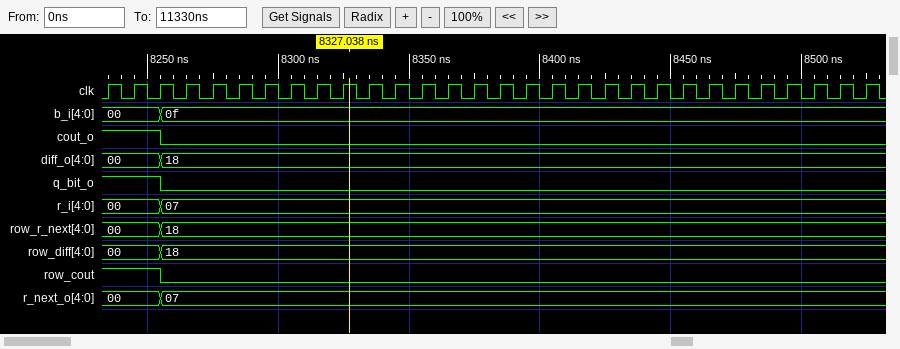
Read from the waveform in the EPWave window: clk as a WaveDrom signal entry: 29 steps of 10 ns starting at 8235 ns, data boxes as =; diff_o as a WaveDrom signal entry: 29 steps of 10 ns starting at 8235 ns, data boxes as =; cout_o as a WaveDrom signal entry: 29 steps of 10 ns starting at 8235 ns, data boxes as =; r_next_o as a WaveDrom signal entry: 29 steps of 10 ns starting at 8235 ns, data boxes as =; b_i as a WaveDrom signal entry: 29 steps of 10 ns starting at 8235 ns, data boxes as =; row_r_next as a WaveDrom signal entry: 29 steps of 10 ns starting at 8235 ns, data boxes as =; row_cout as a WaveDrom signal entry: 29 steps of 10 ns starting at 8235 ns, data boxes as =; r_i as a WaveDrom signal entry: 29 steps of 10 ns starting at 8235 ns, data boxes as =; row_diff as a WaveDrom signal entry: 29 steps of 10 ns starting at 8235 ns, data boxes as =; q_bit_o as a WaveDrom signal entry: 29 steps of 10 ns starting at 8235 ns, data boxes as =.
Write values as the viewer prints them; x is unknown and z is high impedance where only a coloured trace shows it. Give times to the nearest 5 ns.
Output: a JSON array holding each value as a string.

["{name: 'clk', wave: 'p............................'}", "{name: 'diff_o', wave: '=.=..........................', data: '00 18'}", "{name: 'cout_o', wave: '1.0..........................'}", "{name: 'r_next_o', wave: '=.=..........................', data: '00 07'}", "{name: 'b_i', wave: '=.=..........................', data: '00 0f'}", "{name: 'row_r_next', wave: '=.=..........................', data: '00 18'}", "{name: 'row_cout', wave: '1.0..........................'}", "{name: 'r_i', wave: '=.=..........................', data: '00 07'}", "{name: 'row_diff', wave: '=.=..........................', data: '00 18'}", "{name: 'q_bit_o', wave: '1.0..........................'}"]
